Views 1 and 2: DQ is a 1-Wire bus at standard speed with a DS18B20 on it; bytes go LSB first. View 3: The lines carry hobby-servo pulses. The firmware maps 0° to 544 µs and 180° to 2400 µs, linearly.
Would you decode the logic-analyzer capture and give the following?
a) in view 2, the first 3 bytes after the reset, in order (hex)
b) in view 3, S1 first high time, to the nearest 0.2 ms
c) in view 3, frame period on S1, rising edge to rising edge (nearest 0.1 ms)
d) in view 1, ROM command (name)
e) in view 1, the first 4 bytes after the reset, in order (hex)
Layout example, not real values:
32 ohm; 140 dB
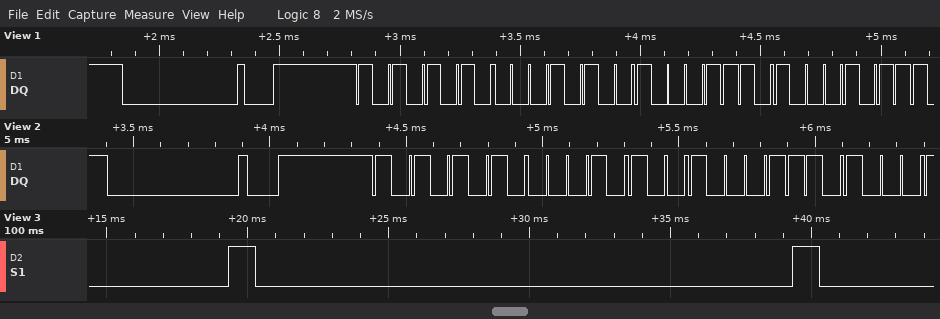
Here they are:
55 28 71; 1.0 ms; 20.0 ms; Match ROM; 55 28 71 D1
